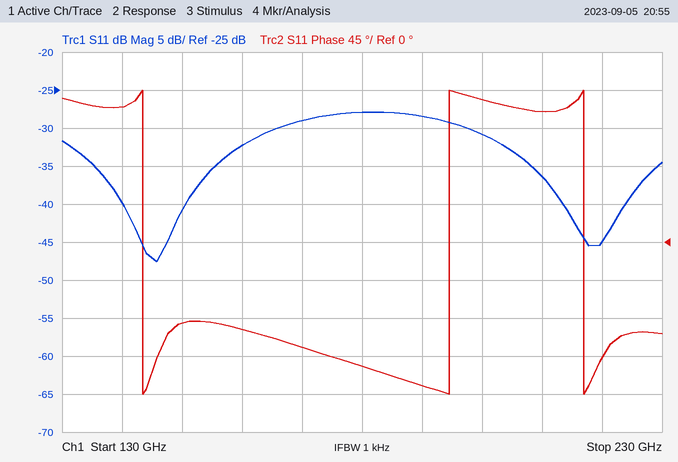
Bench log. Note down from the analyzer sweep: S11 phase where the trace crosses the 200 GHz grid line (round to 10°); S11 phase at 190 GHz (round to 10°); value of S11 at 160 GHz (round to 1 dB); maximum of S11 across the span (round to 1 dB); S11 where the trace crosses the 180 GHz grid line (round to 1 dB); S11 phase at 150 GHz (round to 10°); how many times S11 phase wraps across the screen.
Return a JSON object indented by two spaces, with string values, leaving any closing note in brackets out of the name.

{
  "S11 phase where the trace crosses the 200 GHz grid line": "170°",
  "S11 phase at 190 GHz": "-170°",
  "value of S11 at 160 GHz": "-32 dB",
  "maximum of S11 across the span": "-28 dB",
  "S11 where the trace crosses the 180 GHz grid line": "-28 dB",
  "S11 phase at 150 GHz": "-100°",
  "how many times S11 phase wraps across the screen": "3"
}
